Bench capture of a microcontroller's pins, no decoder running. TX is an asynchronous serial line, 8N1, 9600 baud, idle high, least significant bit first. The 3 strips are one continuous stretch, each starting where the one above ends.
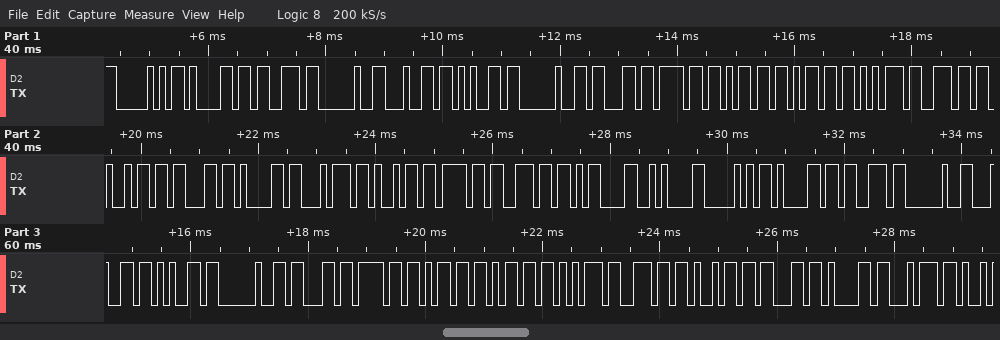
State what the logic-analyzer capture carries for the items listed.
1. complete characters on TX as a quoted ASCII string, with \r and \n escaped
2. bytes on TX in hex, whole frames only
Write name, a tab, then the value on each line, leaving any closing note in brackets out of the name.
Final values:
complete characters on TX as a quoted ASCII string, with \r and \n escaped	"Pas de communication\r\nPas de communicat"
bytes on TX in hex, whole frames only	50 61 73 20 64 65 20 63 6F 6D 6D 75 6E 69 63 61 74 69 6F 6E 0D 0A 50 61 73 20 64 65 20 63 6F 6D 6D 75 6E 69 63 61 74
